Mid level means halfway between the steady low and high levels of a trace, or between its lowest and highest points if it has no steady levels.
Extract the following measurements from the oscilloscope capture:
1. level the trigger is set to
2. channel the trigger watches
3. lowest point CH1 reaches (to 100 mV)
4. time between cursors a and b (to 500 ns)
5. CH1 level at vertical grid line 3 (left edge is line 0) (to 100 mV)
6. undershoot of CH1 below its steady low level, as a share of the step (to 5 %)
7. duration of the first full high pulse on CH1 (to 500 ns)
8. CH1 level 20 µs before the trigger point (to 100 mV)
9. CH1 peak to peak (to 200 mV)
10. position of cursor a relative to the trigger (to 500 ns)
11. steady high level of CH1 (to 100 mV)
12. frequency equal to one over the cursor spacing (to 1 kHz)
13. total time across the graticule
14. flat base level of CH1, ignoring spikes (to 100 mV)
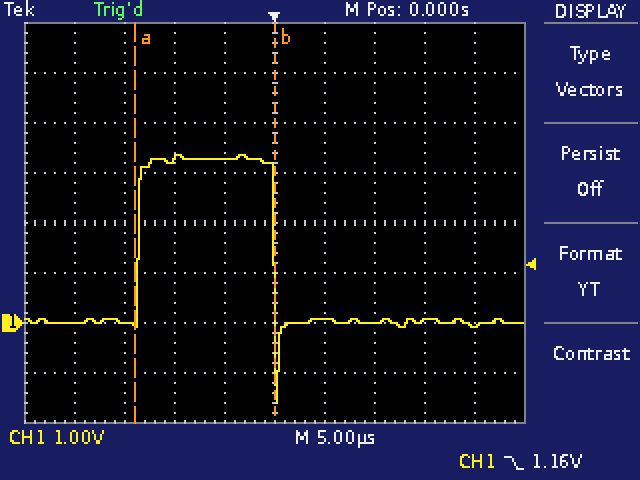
1.16 V
CH1
-1.6 V
14.0 µs
3.3 V
50 %
13.5 µs
0.0 V
5.0 V
-14.0 µs
3.3 V
71 kHz
50 µs
0.0 V
